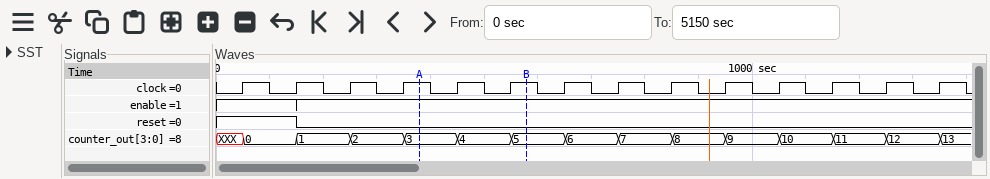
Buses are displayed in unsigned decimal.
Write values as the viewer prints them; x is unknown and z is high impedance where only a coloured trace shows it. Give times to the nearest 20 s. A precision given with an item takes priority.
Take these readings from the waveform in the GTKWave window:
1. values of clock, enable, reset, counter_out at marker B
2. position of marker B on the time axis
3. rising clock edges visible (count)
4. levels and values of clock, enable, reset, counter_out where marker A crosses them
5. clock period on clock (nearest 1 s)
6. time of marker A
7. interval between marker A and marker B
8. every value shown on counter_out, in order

clock=1, enable=1, reset=0, counter_out=5
580 s
14
clock=1, enable=1, reset=0, counter_out=3
100 s
380 s
200 s
XXX, 0, 1, 2, 3, 4, 5, 6, 7, 8, 9, 10, 11, 12, 13
